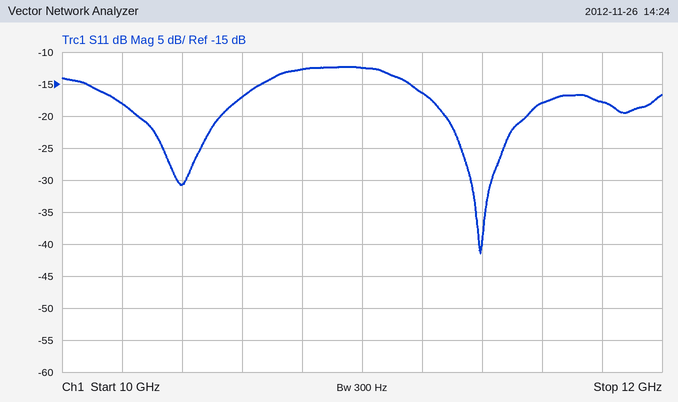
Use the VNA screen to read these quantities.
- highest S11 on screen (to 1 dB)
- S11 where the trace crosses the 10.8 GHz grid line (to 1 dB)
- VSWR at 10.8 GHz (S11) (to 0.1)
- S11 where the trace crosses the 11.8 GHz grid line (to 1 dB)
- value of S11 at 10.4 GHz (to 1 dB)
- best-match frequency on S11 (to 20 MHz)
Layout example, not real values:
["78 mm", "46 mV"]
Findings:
["-12 dB", "-13 dB", "1.6", "-18 dB", "-31 dB", "11.40 GHz"]
